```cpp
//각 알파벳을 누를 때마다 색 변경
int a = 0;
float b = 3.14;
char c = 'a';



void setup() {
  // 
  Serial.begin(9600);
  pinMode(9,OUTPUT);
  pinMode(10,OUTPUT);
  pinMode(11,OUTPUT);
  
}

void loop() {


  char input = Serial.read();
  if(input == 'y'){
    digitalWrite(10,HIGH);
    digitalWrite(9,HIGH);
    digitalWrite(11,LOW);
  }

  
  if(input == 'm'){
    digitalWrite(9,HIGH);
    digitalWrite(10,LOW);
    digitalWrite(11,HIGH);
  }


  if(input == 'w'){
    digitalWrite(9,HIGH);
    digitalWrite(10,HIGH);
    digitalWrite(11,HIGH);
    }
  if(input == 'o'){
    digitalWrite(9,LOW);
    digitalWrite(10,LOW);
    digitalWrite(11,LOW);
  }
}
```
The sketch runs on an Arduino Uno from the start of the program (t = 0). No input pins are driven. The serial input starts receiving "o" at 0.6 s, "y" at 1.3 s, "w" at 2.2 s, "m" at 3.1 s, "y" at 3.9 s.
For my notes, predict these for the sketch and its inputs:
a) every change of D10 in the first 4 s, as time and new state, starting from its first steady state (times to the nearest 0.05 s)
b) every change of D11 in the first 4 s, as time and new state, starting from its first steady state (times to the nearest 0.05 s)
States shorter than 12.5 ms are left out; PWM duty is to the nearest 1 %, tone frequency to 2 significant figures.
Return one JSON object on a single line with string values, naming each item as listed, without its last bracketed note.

{"every change of D10 in the first 4 s, as time and new state, starting from its first steady state": "0 s low; 1.3 s high; 3.1 s low; 3.9 s high", "every change of D11 in the first 4 s, as time and new state, starting from its first steady state": "0 s low; 2.2 s high; 3.9 s low"}
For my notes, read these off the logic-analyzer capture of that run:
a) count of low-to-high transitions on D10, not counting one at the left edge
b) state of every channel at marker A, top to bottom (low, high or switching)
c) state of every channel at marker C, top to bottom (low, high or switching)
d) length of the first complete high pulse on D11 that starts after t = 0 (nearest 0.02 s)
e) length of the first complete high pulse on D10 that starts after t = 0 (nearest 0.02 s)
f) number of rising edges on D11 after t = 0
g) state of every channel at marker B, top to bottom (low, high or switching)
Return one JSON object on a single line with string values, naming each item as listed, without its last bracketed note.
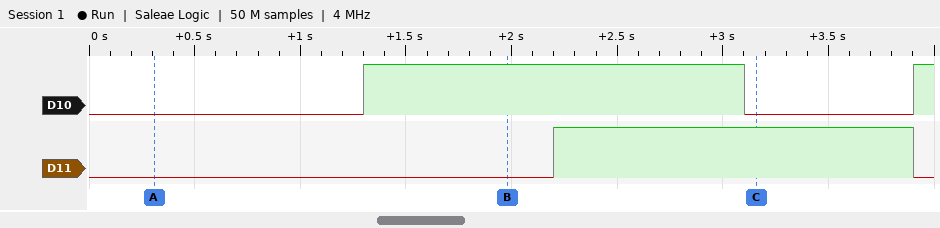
{"count of low-to-high transitions on D10, not counting one at the left edge": "2", "state of every channel at marker A, top to bottom": "D10 low, D11 low", "state of every channel at marker C, top to bottom": "D10 low, D11 high", "length of the first complete high pulse on D11 that starts after t = 0": "1.70 s", "length of the first complete high pulse on D10 that starts after t = 0": "1.80 s", "number of rising edges on D11 after t = 0": "1", "state of every channel at marker B, top to bottom": "D10 high, D11 low"}
